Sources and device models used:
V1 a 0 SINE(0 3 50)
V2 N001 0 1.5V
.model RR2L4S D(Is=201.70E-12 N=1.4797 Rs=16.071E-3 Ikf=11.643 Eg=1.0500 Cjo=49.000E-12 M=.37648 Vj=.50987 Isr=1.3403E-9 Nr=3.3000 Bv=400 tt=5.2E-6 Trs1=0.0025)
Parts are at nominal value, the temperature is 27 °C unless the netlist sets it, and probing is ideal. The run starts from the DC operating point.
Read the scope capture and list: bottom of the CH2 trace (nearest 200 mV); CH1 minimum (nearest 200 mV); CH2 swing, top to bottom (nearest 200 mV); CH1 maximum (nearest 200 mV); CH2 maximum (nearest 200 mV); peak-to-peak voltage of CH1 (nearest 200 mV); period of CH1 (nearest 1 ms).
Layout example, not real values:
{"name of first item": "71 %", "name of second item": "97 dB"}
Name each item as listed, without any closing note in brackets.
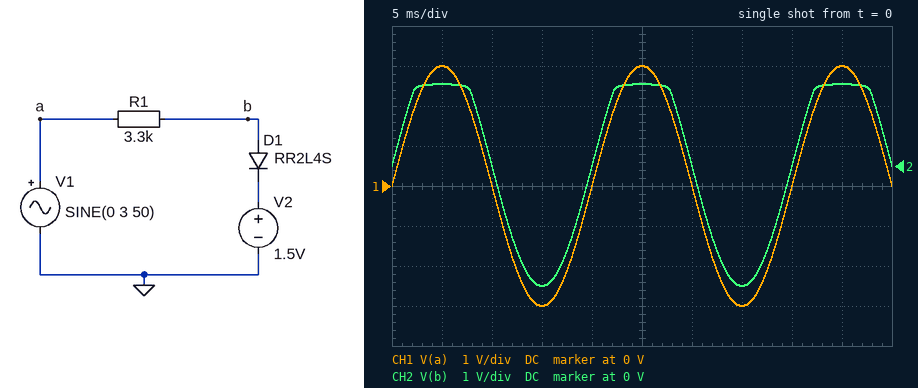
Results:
{"bottom of the CH2 trace": "-3.0 V", "CH1 minimum": "-3.0 V", "CH2 swing, top to bottom": "5.0 V", "CH1 maximum": "3.0 V", "CH2 maximum": "2.0 V", "peak-to-peak voltage of CH1": "6.0 V", "period of CH1": "20 ms"}
